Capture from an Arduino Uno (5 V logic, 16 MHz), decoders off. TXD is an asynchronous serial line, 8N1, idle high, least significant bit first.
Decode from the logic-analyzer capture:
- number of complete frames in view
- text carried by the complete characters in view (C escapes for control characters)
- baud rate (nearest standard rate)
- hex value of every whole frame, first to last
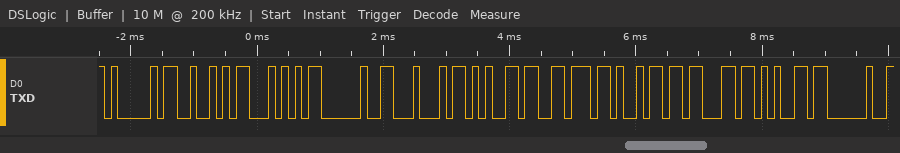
11
"ART Device "
9600 baud
41 52 54 20 44 65 76 69 63 65 20
